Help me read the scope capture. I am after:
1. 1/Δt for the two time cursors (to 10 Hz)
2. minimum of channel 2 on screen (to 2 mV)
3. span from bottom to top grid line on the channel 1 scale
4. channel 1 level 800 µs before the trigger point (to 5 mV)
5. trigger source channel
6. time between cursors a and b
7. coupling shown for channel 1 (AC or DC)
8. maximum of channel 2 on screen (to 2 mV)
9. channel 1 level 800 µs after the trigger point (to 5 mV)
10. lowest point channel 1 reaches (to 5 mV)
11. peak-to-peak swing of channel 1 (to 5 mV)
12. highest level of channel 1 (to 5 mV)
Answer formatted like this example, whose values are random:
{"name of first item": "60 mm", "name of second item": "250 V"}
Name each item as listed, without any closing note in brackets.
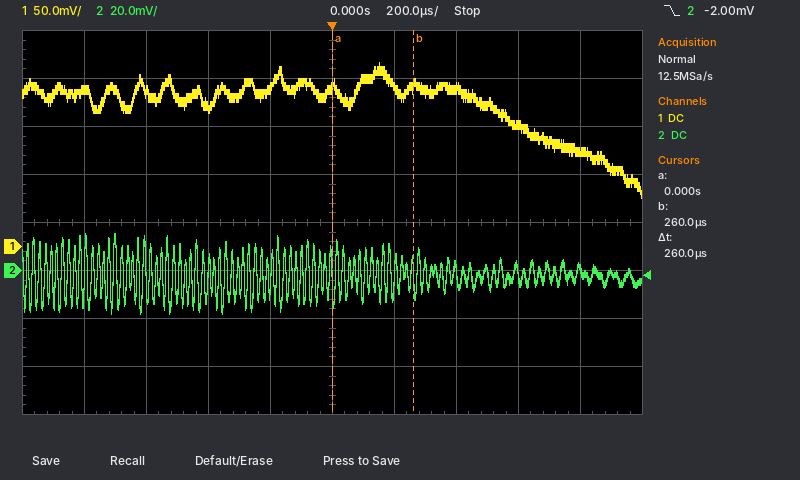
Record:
{"1/Δt for the two time cursors": "3.85 kHz", "minimum of channel 2 on screen": "-18 mV", "span from bottom to top grid line on the channel 1 scale": "400 mV", "channel 1 level 800 µs before the trigger point": "165 mV", "trigger source channel": "channel 2", "time between cursors a and b": "260 µs", "coupling shown for channel 1": "DC", "maximum of channel 2 on screen": "16 mV", "channel 1 level 800 µs after the trigger point": "100 mV", "lowest point channel 1 reaches": "50 mV", "peak-to-peak swing of channel 1": "140 mV", "highest level of channel 1": "190 mV"}
